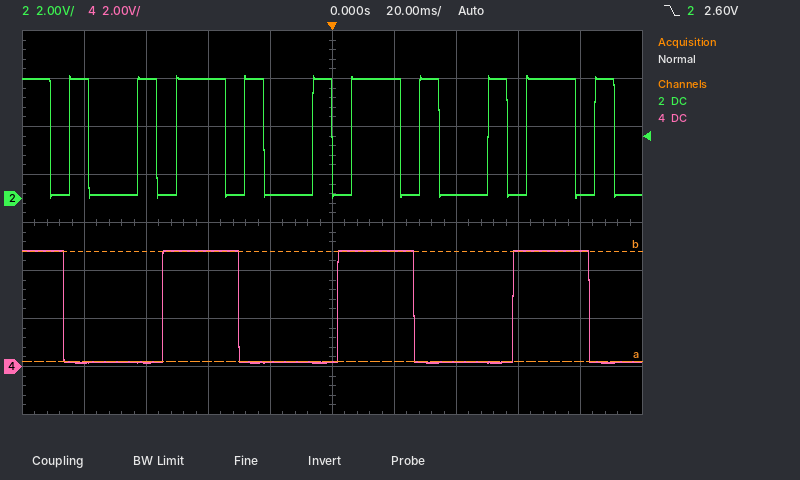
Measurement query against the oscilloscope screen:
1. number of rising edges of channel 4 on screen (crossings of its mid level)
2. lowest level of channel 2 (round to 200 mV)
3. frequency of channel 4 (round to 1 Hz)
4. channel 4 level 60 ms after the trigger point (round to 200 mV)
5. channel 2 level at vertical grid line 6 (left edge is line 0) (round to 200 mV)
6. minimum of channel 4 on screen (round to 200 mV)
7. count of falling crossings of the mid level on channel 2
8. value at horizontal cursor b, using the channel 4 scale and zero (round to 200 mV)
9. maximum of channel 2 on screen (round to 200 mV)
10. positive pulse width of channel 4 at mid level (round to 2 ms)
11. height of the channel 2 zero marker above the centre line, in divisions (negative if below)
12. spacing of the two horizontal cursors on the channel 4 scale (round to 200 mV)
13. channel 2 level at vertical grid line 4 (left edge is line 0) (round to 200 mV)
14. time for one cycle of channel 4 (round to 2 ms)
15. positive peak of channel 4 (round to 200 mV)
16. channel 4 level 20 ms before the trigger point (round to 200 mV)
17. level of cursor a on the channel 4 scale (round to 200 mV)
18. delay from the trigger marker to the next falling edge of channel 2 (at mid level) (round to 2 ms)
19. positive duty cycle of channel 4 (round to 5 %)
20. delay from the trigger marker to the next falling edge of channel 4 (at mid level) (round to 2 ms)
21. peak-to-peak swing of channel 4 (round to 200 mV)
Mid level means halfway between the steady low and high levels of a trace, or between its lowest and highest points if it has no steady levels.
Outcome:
3
0.0 V
18 Hz
4.8 V
5.0 V
200 mV
11
4.8 V
5.2 V
24 ms
+0.5 div
4.6 V
200 mV
56 ms
4.8 V
200 mV
200 mV
22 ms
45 %
26 ms
4.6 V
